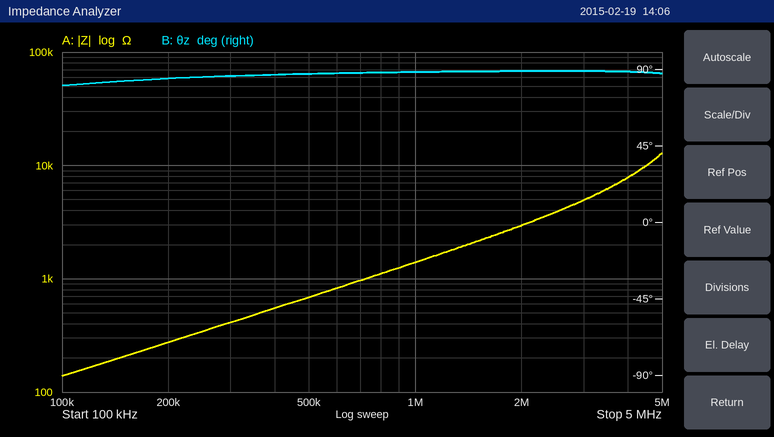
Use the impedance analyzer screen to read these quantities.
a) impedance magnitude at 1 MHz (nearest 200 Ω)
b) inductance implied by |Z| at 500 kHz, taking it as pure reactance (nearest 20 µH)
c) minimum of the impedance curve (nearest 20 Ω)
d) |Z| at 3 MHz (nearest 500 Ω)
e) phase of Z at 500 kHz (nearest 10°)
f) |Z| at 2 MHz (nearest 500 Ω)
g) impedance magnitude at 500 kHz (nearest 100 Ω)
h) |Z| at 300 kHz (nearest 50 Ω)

1.4 kΩ
220 µH
140 Ω
5.0 kΩ
90°
3.0 kΩ
700 Ω
400 Ω
